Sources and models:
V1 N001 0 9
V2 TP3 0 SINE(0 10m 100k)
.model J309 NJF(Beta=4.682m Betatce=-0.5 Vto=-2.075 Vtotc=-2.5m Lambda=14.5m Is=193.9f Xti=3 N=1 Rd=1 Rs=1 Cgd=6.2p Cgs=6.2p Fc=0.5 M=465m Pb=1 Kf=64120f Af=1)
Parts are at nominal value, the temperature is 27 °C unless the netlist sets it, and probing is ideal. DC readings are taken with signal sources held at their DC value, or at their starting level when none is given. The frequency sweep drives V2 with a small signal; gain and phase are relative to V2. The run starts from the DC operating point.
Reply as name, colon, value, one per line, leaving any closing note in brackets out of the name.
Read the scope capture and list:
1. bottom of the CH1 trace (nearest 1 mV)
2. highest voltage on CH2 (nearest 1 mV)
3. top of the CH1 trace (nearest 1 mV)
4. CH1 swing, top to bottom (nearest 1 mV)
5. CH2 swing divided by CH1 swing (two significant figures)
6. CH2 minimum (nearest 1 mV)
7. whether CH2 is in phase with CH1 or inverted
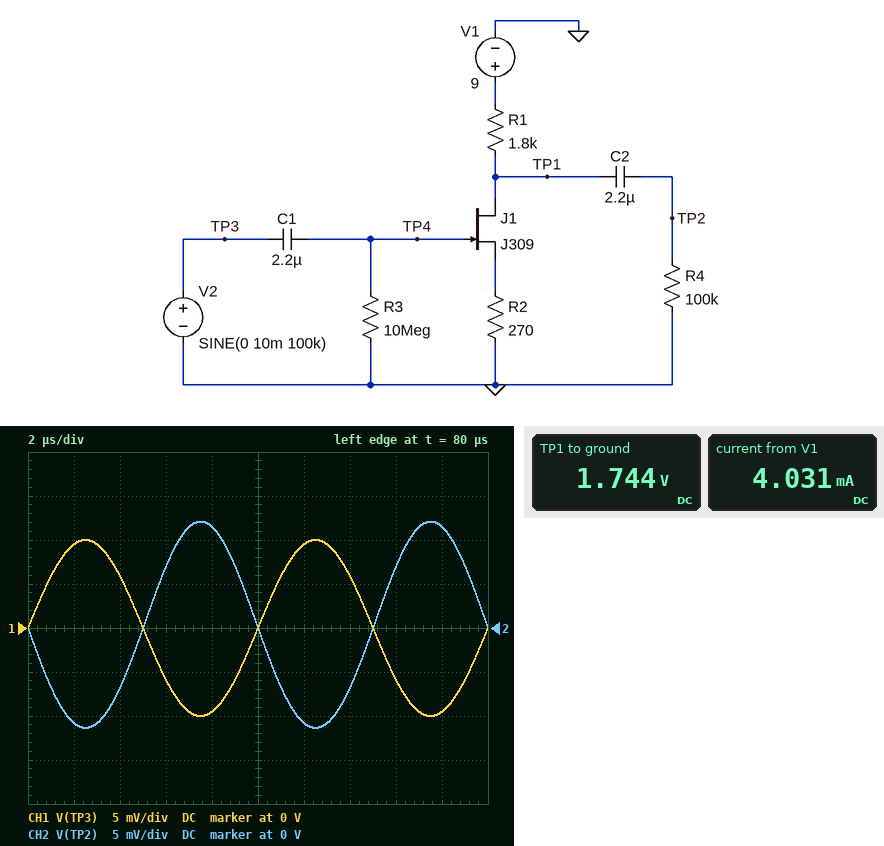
bottom of the CH1 trace: -10 mV
highest voltage on CH2: 12 mV
top of the CH1 trace: 10 mV
CH1 swing, top to bottom: 20 mV
CH2 swing divided by CH1 swing: 1.2
CH2 minimum: -11 mV
whether CH2 is in phase with CH1 or inverted: inverted
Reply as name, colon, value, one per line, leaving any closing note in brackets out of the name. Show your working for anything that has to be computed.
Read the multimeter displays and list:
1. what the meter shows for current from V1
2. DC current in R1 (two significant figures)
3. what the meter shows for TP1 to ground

what the meter shows for current from V1: 4.031 mA
DC current in R1: (9 V - 1.744 V) / 1.8 kΩ = 4.0 mA
what the meter shows for TP1 to ground: 1.744 V
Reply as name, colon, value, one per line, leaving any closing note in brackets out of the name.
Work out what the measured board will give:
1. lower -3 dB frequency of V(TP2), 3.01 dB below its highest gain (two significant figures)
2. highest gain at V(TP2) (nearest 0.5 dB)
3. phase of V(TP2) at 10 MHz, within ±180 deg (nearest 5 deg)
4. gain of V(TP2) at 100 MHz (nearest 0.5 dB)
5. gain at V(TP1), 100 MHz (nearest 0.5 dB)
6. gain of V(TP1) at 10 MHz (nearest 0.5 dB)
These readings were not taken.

lower -3 dB frequency of V(TP2), 3.01 dB below its highest gain: 720 mHz
highest gain at V(TP2): 1.5 dB
phase of V(TP2) at 10 MHz, within ±180 deg: 160 deg
gain of V(TP2) at 100 MHz: 1.0 dB
gain at V(TP1), 100 MHz: 1.0 dB
gain of V(TP1) at 10 MHz: 1.5 dB
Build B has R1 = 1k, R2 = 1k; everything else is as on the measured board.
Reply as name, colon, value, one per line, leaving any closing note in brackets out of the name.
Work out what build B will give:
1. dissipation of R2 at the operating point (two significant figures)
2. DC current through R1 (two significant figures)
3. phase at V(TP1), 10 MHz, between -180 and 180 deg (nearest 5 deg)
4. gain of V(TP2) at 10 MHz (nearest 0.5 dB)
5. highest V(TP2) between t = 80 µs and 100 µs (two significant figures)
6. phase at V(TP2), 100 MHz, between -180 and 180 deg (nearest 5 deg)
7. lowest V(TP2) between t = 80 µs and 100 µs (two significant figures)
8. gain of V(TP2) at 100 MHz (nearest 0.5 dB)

dissipation of R2 at the operating point: 2.3 mW
DC current through R1: 1.5 mA
phase at V(TP1), 10 MHz, between -180 and 180 deg: 160 deg
gain of V(TP2) at 10 MHz: -1.5 dB
highest V(TP2) between t = 80 µs and 100 µs: 8.3 mV
phase at V(TP2), 100 MHz, between -180 and 180 deg: 60 deg
lowest V(TP2) between t = 80 µs and 100 µs: -8.3 mV
gain of V(TP2) at 100 MHz: 0.5 dB
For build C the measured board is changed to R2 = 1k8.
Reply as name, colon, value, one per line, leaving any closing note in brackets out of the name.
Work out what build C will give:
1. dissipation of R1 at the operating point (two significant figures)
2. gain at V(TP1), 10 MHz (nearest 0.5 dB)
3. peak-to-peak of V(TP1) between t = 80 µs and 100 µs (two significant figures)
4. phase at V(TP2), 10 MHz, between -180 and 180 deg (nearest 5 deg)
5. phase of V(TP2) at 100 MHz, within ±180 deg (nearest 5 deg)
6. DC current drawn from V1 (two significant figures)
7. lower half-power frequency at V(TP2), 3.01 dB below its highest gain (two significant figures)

dissipation of R1 at the operating point: 1.5 mW
gain at V(TP1), 10 MHz: -1.0 dB
peak-to-peak of V(TP1) between t = 80 µs and 100 µs: 17 mV
phase at V(TP2), 10 MHz, between -180 and 180 deg: 150 deg
phase of V(TP2) at 100 MHz, within ±180 deg: 35 deg
DC current drawn from V1: 920 µA
lower half-power frequency at V(TP2), 3.01 dB below its highest gain: 1.4 Hz
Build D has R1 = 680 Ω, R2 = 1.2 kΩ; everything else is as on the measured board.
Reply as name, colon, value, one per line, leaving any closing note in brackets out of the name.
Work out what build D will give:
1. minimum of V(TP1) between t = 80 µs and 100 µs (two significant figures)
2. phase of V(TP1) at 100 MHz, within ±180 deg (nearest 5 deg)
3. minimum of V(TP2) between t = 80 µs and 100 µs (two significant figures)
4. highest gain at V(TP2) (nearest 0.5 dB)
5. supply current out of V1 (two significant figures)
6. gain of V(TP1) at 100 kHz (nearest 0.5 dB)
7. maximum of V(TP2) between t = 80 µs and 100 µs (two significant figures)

minimum of V(TP1) between t = 80 µs and 100 µs: 8.1 V
phase of V(TP1) at 100 MHz, within ±180 deg: 70 deg
minimum of V(TP2) between t = 80 µs and 100 µs: -4.8 mV
highest gain at V(TP2): 0 dB
supply current out of V1: 1.3 mA
gain of V(TP1) at 100 kHz: -6.5 dB
maximum of V(TP2) between t = 80 µs and 100 µs: 4.8 mV
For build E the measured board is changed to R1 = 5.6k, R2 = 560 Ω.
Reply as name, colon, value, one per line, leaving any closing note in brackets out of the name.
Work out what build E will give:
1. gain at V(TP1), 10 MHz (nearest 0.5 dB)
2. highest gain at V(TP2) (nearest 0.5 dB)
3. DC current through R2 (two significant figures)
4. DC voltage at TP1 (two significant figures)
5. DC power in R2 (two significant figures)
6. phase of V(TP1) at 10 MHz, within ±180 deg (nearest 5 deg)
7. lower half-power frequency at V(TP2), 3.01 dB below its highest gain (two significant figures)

gain at V(TP1), 10 MHz: -10.0 dB
highest gain at V(TP2): 0 dB
DC current through R2: 1.4 mA
DC voltage at TP1: 940 mV
DC power in R2: 1.2 mW
phase of V(TP1) at 10 MHz, within ±180 deg: 90 deg
lower half-power frequency at V(TP2), 3.01 dB below its highest gain: 31 MHz
